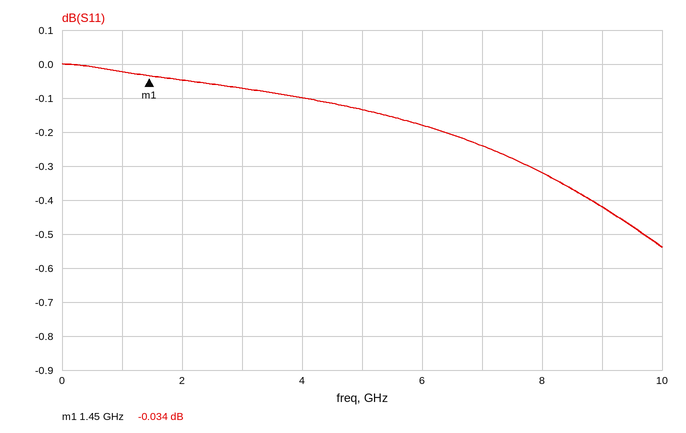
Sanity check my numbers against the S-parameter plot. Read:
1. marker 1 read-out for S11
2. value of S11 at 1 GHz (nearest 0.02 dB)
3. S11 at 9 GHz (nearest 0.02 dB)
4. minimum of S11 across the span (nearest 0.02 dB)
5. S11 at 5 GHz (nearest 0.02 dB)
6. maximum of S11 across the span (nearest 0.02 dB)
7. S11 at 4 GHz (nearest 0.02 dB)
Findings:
-0.034 dB
-0.02 dB
-0.42 dB
-0.54 dB
-0.14 dB
0.00 dB
-0.10 dB
